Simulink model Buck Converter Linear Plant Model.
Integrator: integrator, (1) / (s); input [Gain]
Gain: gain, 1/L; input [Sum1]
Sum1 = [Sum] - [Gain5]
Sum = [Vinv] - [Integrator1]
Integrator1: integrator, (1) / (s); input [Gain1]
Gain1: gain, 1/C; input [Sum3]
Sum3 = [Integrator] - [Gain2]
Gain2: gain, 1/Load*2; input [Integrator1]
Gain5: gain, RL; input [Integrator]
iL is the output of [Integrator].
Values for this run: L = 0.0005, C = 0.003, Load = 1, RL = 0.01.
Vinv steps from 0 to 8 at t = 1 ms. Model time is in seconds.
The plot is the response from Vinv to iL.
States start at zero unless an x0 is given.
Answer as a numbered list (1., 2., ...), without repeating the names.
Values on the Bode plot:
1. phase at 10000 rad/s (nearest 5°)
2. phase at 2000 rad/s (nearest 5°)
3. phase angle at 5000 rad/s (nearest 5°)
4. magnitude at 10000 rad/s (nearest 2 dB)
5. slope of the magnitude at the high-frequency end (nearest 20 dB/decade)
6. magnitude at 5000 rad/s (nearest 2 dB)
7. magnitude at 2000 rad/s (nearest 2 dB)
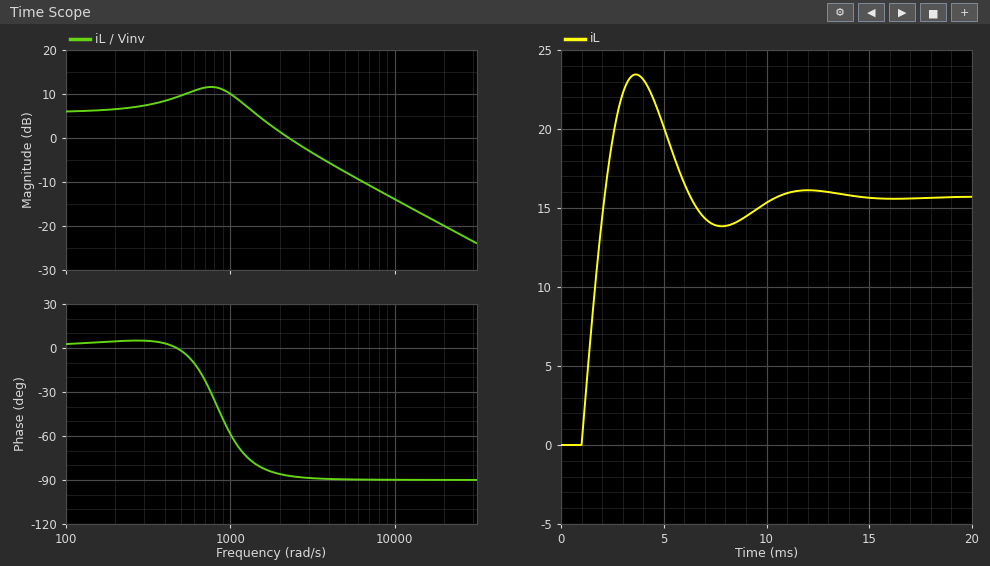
1. -90°
2. -85°
3. -90°
4. -14 dB
5. -20 dB/decade
6. -8 dB
7. 2 dB
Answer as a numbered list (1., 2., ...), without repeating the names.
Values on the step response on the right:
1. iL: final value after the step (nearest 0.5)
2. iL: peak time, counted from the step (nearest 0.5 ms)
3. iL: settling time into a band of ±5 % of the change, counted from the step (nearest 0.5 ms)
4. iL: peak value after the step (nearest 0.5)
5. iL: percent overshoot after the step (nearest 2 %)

1. 15.5
2. 2.5 ms
3. 8.5 ms
4. 23.5
5. 50 %
